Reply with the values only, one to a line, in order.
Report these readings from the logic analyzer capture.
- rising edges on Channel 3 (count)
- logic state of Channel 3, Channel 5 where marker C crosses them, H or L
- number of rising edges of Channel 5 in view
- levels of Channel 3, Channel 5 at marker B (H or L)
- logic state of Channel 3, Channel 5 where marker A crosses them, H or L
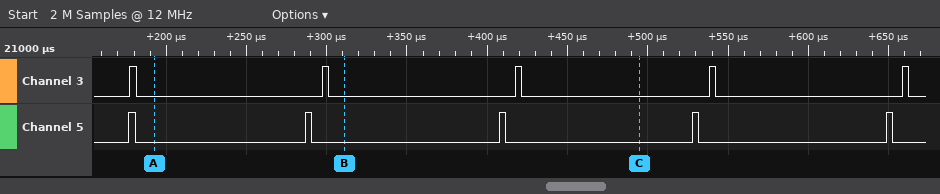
5
Channel 3=L, Channel 5=L
5
Channel 3=L, Channel 5=L
Channel 3=L, Channel 5=L
